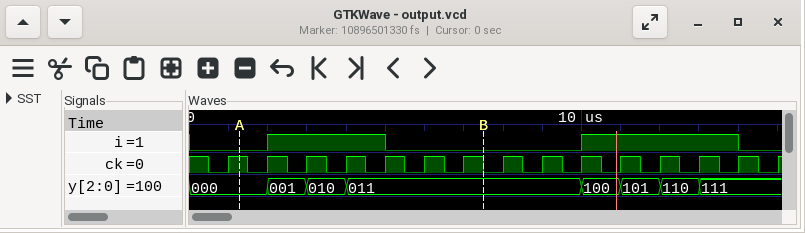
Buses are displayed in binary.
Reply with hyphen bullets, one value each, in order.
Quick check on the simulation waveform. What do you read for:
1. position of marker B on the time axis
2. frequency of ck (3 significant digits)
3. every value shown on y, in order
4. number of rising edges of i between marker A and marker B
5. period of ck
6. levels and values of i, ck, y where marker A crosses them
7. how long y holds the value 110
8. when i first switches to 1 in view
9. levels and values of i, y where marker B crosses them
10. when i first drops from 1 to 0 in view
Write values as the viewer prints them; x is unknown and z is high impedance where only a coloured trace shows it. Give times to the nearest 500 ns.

- 7500 ns
- 1.00 MHz
- 000, 001, 010, 011, 100, 101, 110, 111
- 1
- 1000 ns
- i=0, ck=1, y=000
- 1000 ns
- 2000 ns
- i=0, y=011
- 5000 ns
